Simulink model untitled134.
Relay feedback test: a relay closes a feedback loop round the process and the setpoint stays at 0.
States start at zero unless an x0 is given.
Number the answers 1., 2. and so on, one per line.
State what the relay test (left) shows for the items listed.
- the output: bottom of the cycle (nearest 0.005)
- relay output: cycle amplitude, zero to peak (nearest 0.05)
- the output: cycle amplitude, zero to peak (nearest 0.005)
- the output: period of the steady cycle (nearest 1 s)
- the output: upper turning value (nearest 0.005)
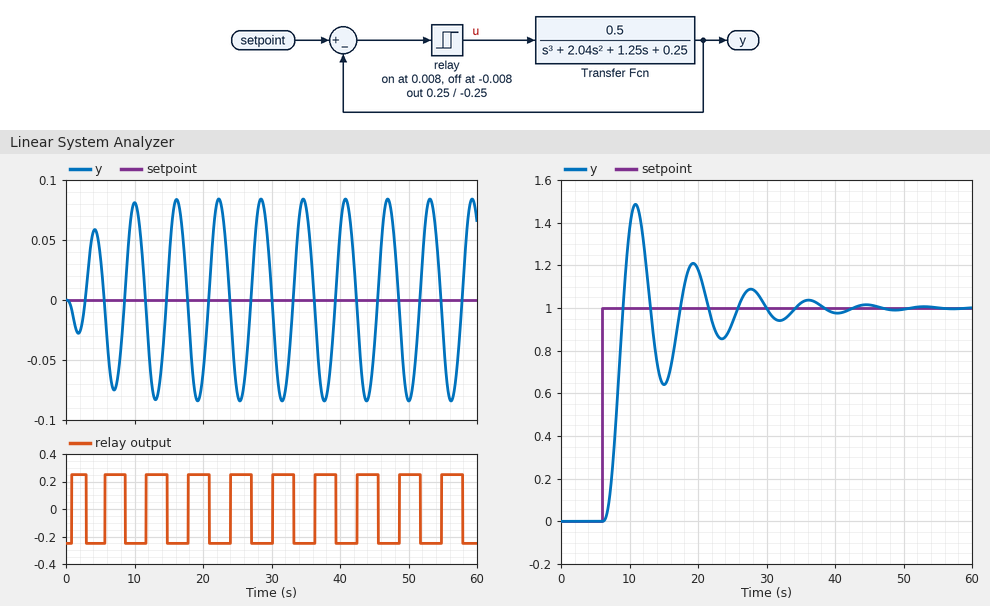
1. -0.085
2. 0.25
3. 0.085
4. 6 s
5. 0.085
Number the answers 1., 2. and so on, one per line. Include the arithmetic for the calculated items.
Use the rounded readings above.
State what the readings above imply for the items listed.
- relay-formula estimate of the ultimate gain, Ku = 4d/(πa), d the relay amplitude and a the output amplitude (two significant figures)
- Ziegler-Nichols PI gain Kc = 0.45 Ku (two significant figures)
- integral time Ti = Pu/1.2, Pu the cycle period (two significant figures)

1. 4 × 0.25 / (π × 0.085) = 3.7
2. 0.45 × 3.7 = 1.7
3. 6 / 1.2 = 5.0 s
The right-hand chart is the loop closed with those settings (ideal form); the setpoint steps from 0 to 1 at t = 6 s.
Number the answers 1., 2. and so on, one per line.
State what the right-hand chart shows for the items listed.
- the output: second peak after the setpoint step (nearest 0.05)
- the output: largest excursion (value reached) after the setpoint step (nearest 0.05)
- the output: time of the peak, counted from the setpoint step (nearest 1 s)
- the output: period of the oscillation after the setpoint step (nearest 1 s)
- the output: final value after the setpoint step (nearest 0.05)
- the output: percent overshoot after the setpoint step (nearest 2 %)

1. 1.20
2. 1.50
3. 5 s
4. 8 s
5. 1.00
6. 48 %
